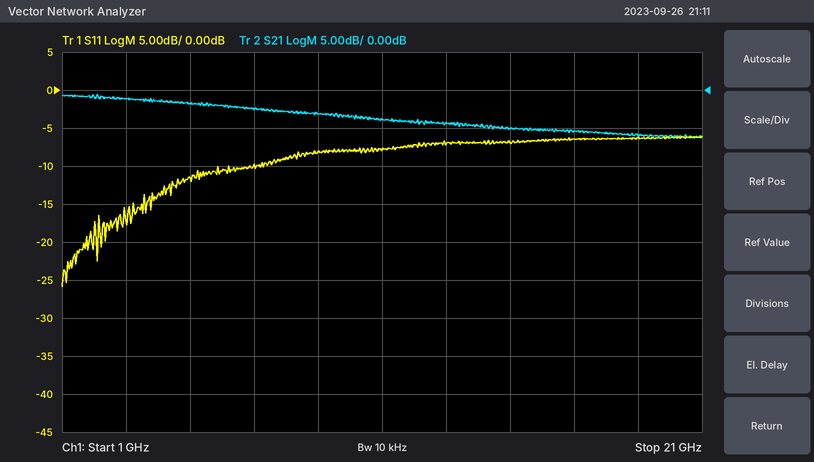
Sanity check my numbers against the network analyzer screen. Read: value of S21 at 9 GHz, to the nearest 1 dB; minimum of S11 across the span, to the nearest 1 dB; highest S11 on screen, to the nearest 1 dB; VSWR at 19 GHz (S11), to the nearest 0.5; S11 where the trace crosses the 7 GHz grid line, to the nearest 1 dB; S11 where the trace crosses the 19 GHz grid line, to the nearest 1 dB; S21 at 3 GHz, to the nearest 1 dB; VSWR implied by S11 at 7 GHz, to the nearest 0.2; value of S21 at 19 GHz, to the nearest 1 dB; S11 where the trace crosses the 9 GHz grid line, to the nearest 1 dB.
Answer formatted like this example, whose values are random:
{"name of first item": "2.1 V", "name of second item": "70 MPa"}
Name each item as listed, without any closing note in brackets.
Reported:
{"value of S21 at 9 GHz, to the nearest 1 dB": "-3 dB", "minimum of S11 across the span, to the nearest 1 dB": "-26 dB", "highest S11 on screen, to the nearest 1 dB": "-6 dB", "VSWR at 19 GHz (S11), to the nearest 0.5": "3.0", "S11 where the trace crosses the 7 GHz grid line, to the nearest 1 dB": "-10 dB", "S11 where the trace crosses the 19 GHz grid line, to the nearest 1 dB": "-6 dB", "S21 at 3 GHz, to the nearest 1 dB": "-1 dB", "VSWR implied by S11 at 7 GHz, to the nearest 0.2": "2.0", "value of S21 at 19 GHz, to the nearest 1 dB": "-6 dB", "S11 where the trace crosses the 9 GHz grid line, to the nearest 1 dB": "-8 dB"}
